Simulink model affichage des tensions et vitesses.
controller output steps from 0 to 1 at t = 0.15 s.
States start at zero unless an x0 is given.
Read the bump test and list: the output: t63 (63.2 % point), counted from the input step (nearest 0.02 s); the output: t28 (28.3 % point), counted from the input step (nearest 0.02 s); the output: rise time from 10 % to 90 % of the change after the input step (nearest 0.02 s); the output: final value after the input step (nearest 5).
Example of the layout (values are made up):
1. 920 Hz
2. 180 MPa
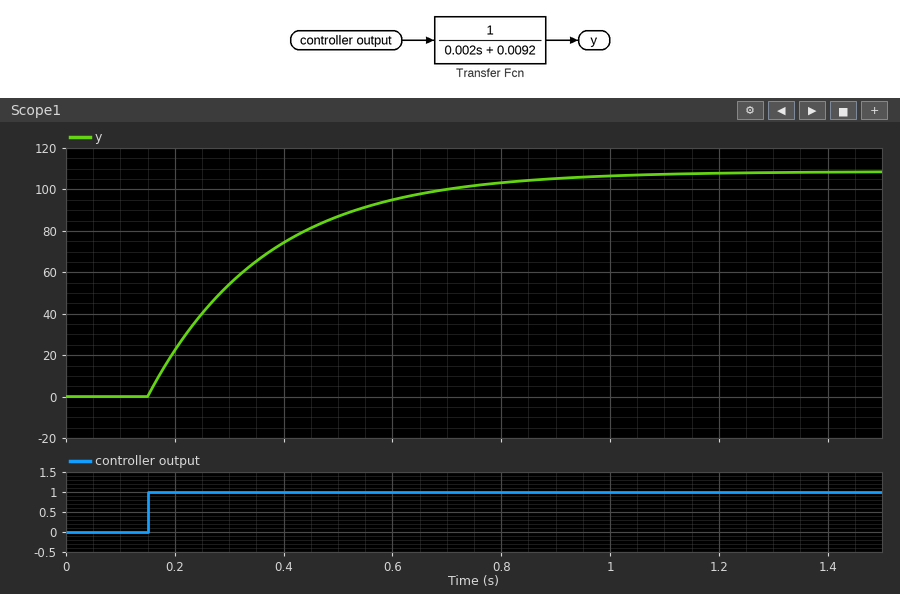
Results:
1. 0.22 s
2. 0.08 s
3. 0.48 s
4. 110
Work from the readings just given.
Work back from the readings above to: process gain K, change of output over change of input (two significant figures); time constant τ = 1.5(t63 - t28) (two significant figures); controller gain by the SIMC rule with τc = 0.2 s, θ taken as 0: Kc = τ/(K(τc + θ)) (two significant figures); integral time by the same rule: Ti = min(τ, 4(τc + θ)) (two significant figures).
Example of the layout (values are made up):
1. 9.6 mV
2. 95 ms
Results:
1. 110
2. 0.21 s
3. 0.0095
4. 0.21 s
